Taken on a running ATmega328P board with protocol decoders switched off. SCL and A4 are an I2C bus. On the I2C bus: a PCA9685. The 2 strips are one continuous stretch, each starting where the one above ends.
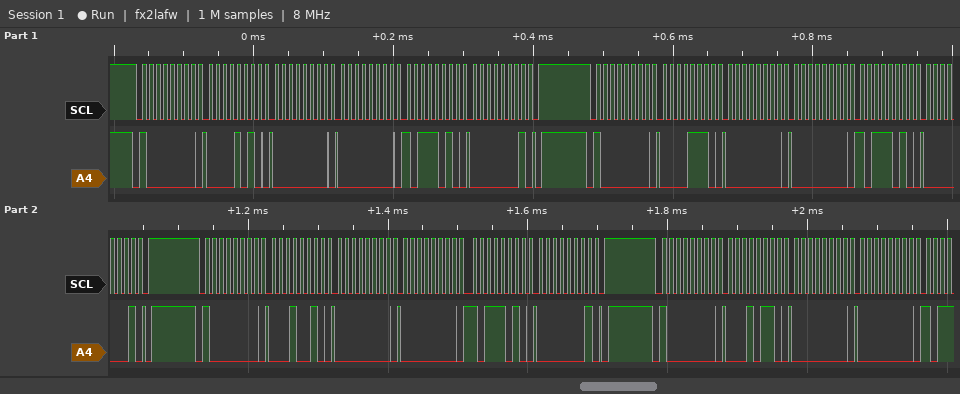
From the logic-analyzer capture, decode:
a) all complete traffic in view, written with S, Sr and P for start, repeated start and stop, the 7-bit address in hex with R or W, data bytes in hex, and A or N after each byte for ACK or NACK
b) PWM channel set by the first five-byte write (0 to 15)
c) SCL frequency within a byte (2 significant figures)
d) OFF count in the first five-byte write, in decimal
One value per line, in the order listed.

S 40W A 0A A 00 A 00 A BA A 01 A P S 40W A 0E A 00 A 00 A BA A 01 A P S 40W A 12 A 00 A 00 A BA A 01 A P S 40W A 16 A 00 A 00 A
1
100 kHz
442
